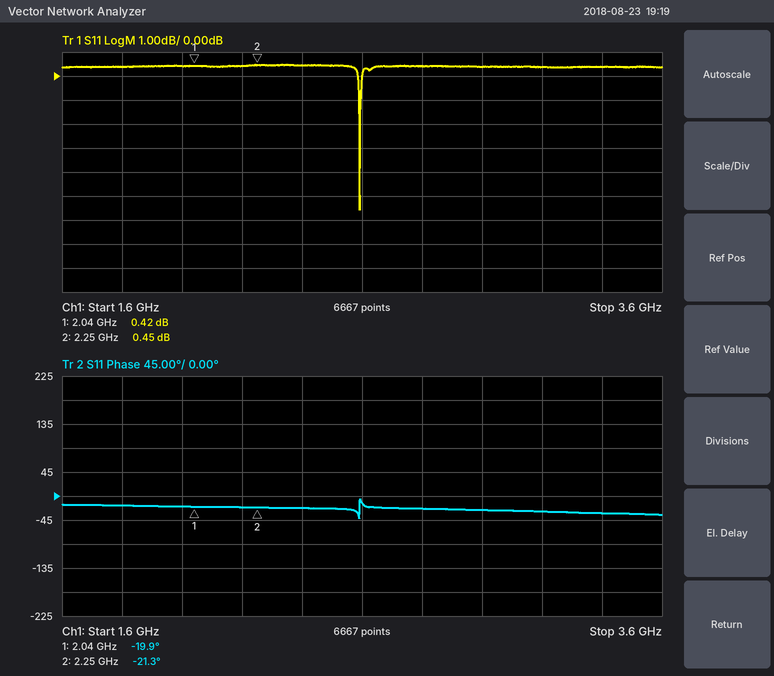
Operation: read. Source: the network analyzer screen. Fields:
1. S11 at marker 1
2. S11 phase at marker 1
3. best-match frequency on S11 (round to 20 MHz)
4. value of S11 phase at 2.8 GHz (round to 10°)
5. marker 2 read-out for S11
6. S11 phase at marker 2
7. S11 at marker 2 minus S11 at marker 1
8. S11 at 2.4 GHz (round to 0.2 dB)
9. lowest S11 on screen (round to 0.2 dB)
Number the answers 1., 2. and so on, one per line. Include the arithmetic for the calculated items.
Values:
1. 0.42 dB
2. -19.9°
3. 2.60 GHz
4. -20°
5. 0.45 dB
6. -21.3°
7. 0.45 − (0.42) = 0.03 dB
8. 0.4 dB
9. -5.6 dB
